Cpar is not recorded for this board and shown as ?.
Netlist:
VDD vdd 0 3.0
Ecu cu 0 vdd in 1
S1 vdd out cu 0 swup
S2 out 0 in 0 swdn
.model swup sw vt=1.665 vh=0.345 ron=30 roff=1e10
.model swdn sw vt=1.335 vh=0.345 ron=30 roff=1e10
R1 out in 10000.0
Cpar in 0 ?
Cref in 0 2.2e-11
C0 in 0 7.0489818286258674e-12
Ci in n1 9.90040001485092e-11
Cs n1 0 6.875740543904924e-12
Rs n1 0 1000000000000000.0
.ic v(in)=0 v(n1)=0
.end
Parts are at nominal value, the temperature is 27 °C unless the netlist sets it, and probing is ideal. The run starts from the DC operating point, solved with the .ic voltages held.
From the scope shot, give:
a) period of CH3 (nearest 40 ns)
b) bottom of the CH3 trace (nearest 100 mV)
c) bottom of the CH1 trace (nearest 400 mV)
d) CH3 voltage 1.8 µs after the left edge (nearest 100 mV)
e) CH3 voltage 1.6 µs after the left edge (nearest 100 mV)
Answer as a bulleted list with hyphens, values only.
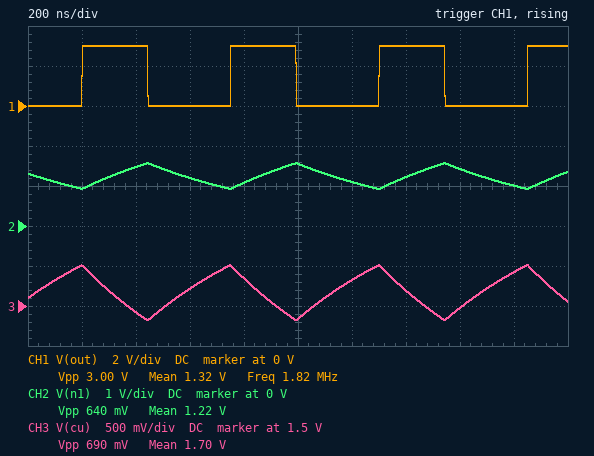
- 560 ns
- 1.3 V
- 0 V
- 1.9 V
- 1.5 V
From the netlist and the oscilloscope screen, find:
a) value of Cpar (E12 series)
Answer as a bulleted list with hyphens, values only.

- 22 pF
